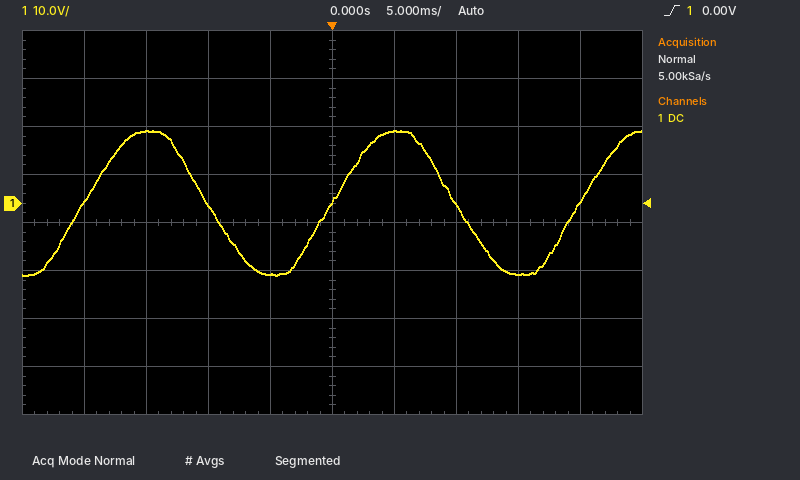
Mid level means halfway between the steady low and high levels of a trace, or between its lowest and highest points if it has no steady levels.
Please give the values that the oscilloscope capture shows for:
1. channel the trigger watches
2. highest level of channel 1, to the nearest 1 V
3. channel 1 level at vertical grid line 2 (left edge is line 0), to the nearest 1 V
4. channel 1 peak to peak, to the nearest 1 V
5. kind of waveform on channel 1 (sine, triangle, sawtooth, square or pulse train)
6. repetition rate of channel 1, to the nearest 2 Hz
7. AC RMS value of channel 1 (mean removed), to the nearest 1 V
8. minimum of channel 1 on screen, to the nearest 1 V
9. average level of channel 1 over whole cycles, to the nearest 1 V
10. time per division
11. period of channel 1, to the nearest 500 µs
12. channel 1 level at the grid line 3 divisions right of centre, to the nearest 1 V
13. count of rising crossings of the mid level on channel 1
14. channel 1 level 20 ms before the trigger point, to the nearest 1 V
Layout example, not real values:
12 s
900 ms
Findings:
channel 1
15 V
15 V
30 V
sine
50 Hz
11 V
-15 V
0 V
5 ms
20.0 ms
-15 V
3
0 V
